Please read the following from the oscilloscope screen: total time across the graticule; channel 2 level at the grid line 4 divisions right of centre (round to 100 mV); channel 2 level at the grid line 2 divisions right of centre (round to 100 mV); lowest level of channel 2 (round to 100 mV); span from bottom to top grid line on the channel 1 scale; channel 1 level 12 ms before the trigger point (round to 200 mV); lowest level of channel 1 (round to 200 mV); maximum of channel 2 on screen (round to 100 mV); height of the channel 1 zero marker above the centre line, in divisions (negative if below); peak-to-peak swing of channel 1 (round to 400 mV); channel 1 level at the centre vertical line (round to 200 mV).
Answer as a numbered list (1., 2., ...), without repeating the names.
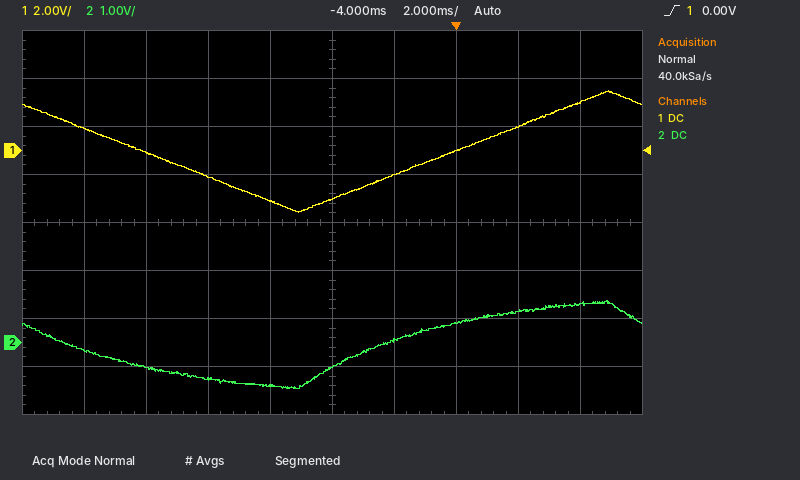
1. 20 ms
2. 800 mV
3. 400 mV
4. -1.0 V
5. 16 V
6. 1.0 V
7. -2.6 V
8. 900 mV
9. +1.5 div
10. 5.2 V
11. -2.0 V
